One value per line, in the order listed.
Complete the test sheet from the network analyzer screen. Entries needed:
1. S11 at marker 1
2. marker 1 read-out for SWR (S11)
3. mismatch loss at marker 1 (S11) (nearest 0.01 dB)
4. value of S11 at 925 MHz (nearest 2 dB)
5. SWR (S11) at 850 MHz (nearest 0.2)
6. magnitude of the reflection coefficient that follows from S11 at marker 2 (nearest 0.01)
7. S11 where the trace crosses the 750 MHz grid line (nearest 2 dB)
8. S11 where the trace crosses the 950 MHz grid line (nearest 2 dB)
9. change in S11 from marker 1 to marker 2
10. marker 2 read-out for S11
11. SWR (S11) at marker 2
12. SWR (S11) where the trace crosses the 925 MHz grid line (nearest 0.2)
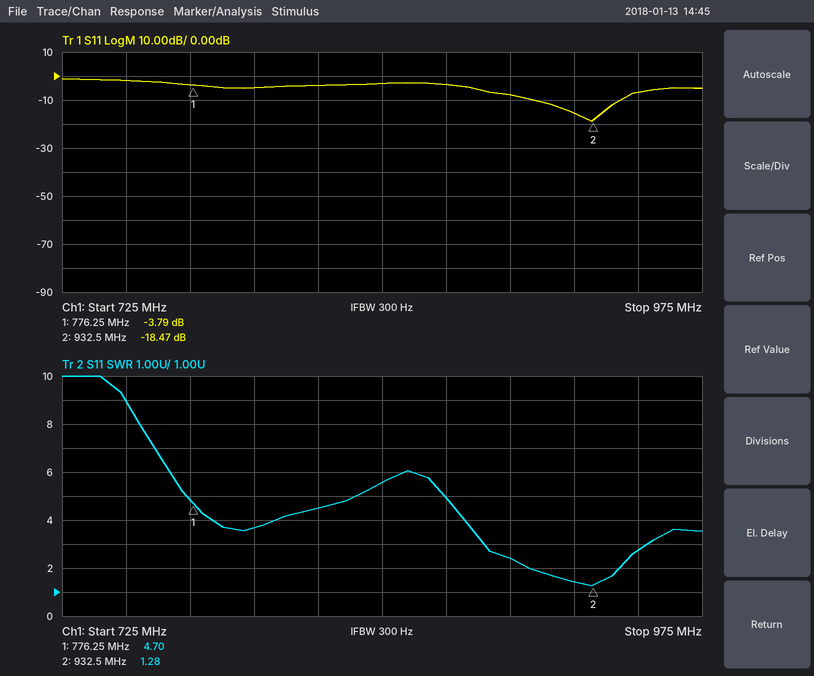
-3.79 dB
4.70
2.35 dB
-16 dB
5.6
0.12
-2 dB
-6 dB
-14.68 dB
-18.47 dB
1.28
1.4
